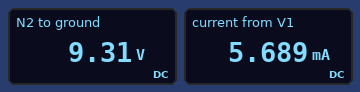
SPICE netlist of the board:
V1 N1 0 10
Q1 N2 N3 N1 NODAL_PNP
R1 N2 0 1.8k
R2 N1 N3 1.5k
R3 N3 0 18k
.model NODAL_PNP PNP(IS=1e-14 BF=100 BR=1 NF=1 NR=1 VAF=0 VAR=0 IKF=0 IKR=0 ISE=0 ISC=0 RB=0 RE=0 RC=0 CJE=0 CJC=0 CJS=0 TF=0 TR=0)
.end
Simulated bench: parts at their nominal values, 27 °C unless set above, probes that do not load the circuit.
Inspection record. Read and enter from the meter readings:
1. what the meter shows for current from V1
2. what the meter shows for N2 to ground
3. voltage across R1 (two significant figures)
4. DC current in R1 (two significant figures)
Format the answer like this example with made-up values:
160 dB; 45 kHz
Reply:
5.689 mA; 9.31 V; 9.3 V; 5.2 mA
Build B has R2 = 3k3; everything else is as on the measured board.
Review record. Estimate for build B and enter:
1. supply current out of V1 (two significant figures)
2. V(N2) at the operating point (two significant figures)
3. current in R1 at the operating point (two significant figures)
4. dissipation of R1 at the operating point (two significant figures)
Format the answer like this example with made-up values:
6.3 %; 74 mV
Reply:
6.0 mA; 9.9 V; 5.5 mA; 55 mW
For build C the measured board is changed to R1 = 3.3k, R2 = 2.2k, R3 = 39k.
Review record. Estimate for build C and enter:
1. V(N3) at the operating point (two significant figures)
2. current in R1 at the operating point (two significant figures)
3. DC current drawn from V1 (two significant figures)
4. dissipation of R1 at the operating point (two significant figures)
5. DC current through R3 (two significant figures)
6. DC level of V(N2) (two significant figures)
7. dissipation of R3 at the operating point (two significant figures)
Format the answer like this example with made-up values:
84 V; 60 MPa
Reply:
9.5 V; 9.2 µA; 250 µA; 280 nW; 240 µA; 30 mV; 2.3 mW
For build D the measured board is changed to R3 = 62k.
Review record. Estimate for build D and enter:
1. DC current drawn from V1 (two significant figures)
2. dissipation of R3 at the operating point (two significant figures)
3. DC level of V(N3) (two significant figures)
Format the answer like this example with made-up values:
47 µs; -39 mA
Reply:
160 µA; 1.5 mW; 9.8 V
